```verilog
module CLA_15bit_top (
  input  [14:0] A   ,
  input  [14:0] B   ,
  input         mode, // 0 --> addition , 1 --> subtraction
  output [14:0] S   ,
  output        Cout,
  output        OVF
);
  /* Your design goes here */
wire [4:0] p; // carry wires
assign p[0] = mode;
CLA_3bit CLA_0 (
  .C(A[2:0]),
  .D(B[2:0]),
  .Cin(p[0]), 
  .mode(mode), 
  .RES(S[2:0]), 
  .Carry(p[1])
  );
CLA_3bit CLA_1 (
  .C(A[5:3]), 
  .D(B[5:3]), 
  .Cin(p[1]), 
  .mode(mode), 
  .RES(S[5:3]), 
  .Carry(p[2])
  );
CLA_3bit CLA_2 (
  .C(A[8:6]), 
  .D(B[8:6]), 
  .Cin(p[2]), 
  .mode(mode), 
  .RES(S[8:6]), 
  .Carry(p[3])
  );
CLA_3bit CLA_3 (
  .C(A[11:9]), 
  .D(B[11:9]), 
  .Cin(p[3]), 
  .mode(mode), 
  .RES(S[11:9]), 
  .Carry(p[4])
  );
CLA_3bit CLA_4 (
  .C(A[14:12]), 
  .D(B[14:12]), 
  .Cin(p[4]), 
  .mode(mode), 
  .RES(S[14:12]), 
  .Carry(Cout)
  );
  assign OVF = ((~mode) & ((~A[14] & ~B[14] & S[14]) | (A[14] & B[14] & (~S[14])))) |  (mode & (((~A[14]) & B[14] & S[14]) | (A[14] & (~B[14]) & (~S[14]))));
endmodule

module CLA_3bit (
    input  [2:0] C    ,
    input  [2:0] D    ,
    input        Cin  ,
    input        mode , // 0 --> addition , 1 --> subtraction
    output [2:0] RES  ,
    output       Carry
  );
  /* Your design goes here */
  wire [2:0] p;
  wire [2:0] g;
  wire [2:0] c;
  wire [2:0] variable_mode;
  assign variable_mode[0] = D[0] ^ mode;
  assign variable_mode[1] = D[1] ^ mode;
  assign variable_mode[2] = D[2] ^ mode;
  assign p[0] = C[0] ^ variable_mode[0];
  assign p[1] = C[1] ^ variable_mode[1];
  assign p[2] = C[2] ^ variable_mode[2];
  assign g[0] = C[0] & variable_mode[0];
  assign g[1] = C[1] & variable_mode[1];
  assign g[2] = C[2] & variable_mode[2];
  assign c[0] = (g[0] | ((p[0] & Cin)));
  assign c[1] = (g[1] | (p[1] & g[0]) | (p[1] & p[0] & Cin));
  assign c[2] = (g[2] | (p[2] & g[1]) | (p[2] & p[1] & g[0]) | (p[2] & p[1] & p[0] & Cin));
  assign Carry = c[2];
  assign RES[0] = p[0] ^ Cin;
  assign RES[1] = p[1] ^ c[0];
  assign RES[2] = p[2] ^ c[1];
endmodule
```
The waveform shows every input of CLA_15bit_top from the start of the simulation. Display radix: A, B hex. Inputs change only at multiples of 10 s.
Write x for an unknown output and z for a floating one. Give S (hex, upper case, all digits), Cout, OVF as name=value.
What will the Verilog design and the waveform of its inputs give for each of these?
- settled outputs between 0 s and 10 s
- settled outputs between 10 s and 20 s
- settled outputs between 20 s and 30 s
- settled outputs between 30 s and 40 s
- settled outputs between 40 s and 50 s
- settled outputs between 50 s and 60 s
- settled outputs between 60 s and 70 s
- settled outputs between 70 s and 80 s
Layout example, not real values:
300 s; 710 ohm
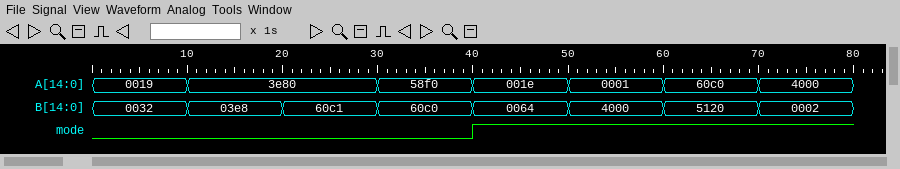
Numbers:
S=004B, Cout=0, OVF=0; S=4268, Cout=0, OVF=1; S=1F41, Cout=1, OVF=0; S=39B0, Cout=1, OVF=1; S=7FBA, Cout=0, OVF=0; S=4001, Cout=0, OVF=1; S=0FA0, Cout=1, OVF=0; S=3FFE, Cout=1, OVF=1
